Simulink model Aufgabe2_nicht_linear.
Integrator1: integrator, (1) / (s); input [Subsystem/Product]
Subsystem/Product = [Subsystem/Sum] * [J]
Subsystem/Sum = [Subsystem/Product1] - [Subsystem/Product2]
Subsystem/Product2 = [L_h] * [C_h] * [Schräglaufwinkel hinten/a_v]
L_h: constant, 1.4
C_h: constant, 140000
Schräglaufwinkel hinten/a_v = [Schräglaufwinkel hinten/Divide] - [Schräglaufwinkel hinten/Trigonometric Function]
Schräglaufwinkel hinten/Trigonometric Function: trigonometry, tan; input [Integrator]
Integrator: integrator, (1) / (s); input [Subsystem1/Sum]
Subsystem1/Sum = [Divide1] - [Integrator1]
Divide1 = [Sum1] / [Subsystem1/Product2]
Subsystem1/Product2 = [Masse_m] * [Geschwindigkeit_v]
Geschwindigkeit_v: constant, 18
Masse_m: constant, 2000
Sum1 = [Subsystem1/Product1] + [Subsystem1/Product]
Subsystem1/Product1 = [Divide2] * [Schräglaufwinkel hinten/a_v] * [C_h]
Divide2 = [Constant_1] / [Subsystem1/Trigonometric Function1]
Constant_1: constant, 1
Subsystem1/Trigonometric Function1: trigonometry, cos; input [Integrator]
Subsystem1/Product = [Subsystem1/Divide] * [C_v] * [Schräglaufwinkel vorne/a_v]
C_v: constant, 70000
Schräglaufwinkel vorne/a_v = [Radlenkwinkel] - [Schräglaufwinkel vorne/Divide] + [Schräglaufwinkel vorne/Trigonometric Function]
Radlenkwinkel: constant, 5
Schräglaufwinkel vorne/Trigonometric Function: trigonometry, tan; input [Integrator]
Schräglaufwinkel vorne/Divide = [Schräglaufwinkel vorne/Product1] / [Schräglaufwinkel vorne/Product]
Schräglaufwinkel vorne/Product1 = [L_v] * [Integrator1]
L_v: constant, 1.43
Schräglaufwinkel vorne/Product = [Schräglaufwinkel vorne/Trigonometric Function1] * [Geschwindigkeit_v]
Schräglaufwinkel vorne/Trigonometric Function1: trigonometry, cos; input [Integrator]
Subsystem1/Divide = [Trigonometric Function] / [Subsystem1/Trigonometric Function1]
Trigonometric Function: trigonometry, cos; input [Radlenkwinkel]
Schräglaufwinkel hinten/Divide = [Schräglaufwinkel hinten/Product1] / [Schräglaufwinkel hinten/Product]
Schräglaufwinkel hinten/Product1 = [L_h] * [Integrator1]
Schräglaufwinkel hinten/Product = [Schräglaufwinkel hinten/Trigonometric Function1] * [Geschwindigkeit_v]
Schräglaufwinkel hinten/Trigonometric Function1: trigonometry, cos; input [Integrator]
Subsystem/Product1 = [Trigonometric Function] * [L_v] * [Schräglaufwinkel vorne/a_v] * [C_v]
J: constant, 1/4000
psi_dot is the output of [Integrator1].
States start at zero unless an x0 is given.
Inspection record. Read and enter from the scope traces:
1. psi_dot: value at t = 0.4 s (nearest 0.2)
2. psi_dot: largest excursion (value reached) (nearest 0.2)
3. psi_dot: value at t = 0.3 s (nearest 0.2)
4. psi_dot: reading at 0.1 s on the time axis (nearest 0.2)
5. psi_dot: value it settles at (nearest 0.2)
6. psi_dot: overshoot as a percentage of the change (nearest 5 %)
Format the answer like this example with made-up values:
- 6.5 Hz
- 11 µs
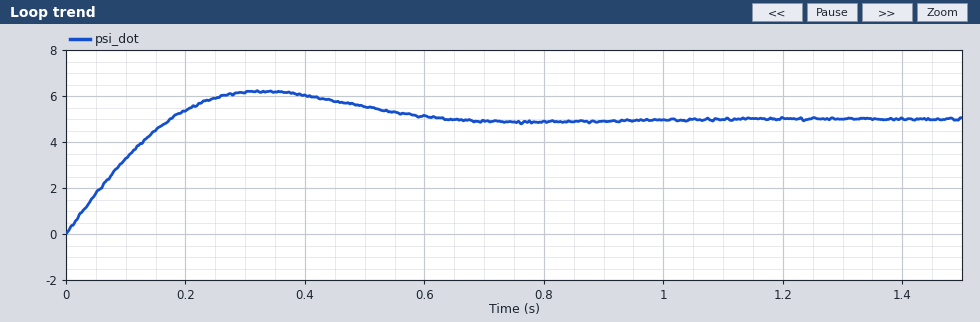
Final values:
- 6.0
- 6.2
- 6.2
- 3.2
- 5.0
- 25 %
